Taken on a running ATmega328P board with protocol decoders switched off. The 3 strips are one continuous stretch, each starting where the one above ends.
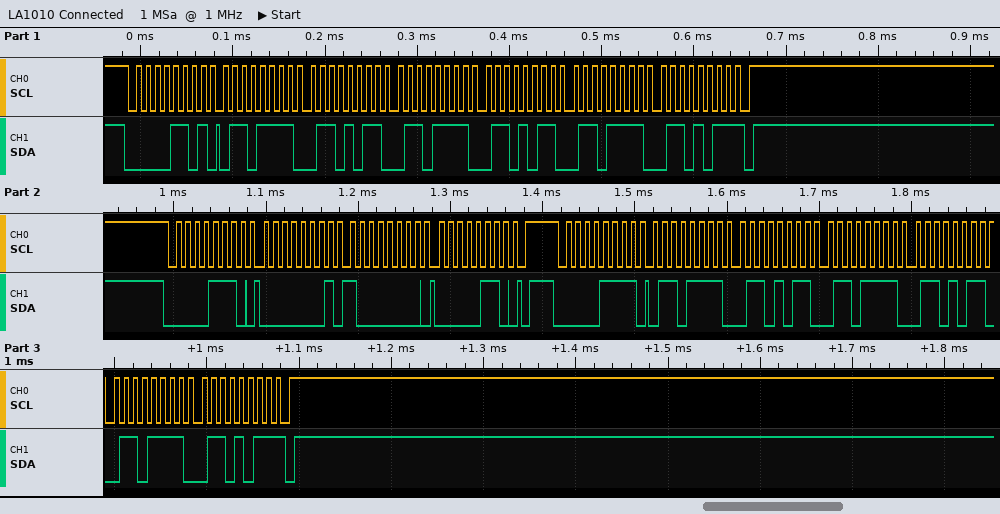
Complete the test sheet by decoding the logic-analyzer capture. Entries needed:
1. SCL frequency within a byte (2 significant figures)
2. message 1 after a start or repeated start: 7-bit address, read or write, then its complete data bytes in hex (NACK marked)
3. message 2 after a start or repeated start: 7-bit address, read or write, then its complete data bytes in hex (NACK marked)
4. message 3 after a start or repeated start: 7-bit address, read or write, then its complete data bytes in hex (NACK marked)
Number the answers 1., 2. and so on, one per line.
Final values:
1. 100 kHz
2. 0x06 read: 6F 6B 6F 6B 6F 6B NACK
3. 0x07 write: 01 80 06
4. 0x07 read: 6F 6B 6F 6B 6F 6B NACK
